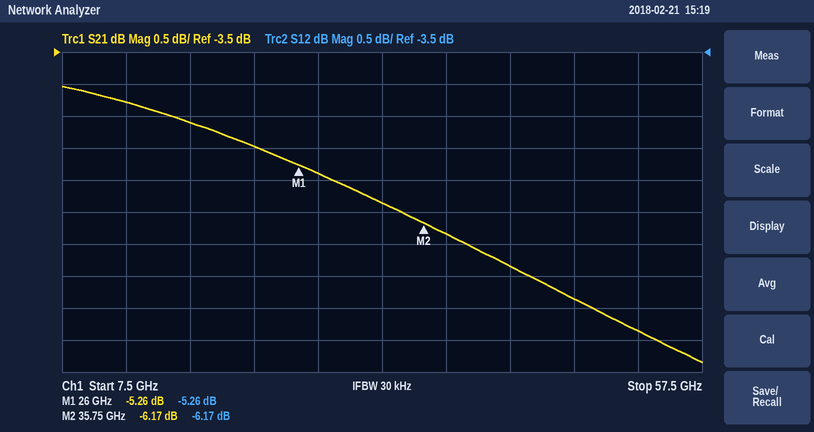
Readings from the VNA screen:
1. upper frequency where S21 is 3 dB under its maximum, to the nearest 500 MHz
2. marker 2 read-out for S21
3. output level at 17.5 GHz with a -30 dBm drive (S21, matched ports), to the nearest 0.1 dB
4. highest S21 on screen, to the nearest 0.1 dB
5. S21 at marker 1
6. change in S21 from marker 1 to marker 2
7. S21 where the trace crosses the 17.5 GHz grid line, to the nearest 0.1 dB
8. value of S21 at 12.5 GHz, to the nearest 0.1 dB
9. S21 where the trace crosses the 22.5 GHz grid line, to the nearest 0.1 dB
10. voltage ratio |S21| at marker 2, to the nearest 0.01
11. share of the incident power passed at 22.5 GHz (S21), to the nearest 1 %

44.5 GHz
-6.17 dB
-34.6 dBm
-4.0 dB
-5.26 dB
-0.91 dB
-4.6 dB
-4.3 dB
-5.0 dB
0.49
32 %
